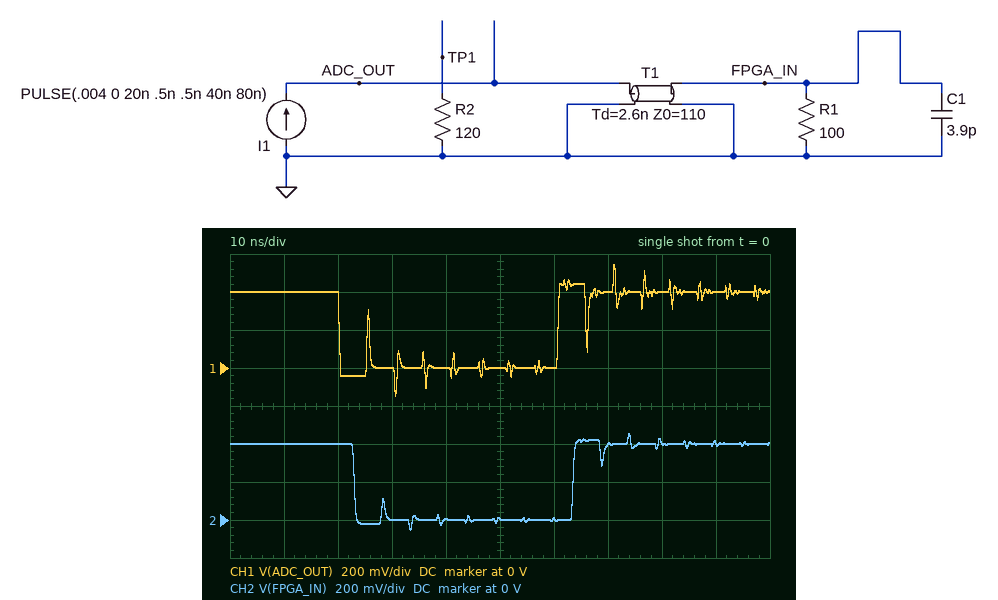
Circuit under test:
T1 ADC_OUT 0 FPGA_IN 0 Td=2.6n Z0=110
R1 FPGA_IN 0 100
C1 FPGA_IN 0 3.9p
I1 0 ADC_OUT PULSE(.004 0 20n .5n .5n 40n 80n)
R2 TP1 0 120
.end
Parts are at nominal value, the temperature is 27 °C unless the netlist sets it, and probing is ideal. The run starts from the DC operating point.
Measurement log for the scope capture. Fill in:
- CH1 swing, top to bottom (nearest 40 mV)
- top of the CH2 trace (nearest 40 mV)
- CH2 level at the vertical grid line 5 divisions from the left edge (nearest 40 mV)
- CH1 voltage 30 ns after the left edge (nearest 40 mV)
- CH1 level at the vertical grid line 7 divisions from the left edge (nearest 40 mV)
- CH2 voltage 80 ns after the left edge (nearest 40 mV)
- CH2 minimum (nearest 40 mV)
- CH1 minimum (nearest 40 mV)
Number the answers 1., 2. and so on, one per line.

1. 680 mV
2. 440 mV
3. 0 V
4. 0 V
5. 400 mV
6. 400 mV
7. -40 mV
8. -160 mV
